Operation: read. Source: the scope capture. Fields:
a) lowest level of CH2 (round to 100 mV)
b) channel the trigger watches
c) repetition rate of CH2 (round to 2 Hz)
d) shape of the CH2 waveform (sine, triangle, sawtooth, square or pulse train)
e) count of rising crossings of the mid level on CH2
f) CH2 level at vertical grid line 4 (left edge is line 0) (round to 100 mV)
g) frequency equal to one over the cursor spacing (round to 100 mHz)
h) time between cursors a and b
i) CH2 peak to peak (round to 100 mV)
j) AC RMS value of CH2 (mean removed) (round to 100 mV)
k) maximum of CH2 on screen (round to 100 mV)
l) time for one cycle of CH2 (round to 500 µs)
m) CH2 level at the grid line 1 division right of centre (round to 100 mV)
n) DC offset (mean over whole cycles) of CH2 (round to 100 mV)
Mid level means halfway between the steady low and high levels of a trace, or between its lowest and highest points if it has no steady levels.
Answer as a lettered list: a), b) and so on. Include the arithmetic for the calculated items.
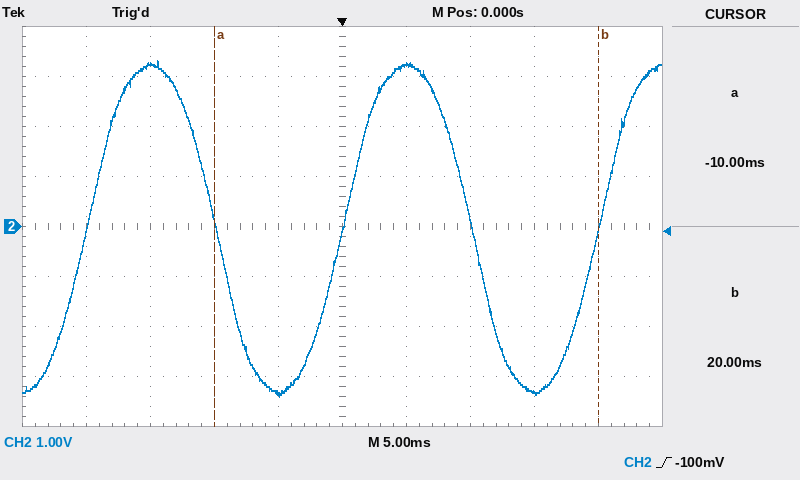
a) -3.4 V
b) CH2
c) 1 / 20.0 ms ≈ 50 Hz
d) sine
e) 3
f) -3.3 V
g) 1 / 30.0 ms ≈ 33.3 Hz
h) 20 ms − (-10 ms) = 30.0 ms
i) 3.3 V − (-3.4 V) = 6.7 V
j) 6.7 V / (2√2) ≈ 2.4 V
k) 3.3 V
l) 20.0 ms
m) 3.2 V
n) (3.3 V + (-3.4 V)) / 2 ≈ 0.0 V
